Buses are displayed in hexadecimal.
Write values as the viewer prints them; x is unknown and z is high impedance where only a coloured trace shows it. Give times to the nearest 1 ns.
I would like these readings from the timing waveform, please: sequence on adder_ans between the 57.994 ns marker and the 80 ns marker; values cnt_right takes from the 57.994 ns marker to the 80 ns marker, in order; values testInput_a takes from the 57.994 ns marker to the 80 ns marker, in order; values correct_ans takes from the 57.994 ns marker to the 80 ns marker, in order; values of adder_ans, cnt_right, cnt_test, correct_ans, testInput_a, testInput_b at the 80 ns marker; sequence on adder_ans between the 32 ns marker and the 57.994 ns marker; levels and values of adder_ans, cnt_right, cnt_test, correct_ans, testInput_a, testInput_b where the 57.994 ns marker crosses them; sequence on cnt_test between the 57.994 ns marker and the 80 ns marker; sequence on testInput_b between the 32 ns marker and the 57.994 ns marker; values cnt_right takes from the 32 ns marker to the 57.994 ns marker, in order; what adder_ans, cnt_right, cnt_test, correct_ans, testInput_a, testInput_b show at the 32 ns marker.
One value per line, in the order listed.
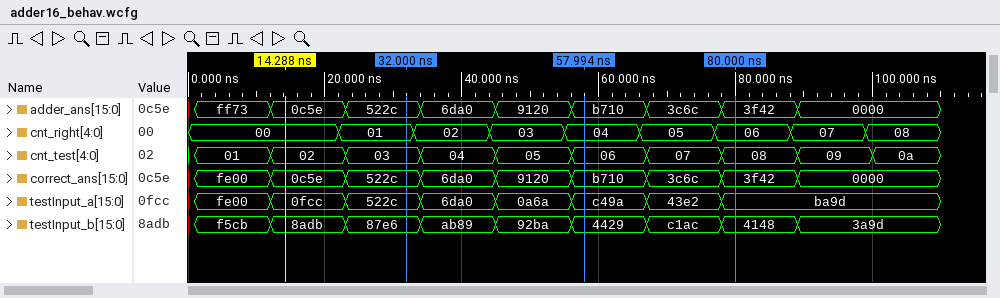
b710, 3c6c, 3f42
04, 05, 06
c49a, 43e2, ba9d
b710, 3c6c, 3f42
adder_ans=3f42, cnt_right=06, cnt_test=08, correct_ans=3f42, testInput_a=ba9d, testInput_b=4148
522c, 6da0, 9120, b710
adder_ans=b710, cnt_right=04, cnt_test=06, correct_ans=b710, testInput_a=c49a, testInput_b=4429
06, 07, 08
87e6, ab89, 92ba, 4429
01, 02, 03, 04
adder_ans=522c, cnt_right=01, cnt_test=03, correct_ans=522c, testInput_a=522c, testInput_b=87e6
